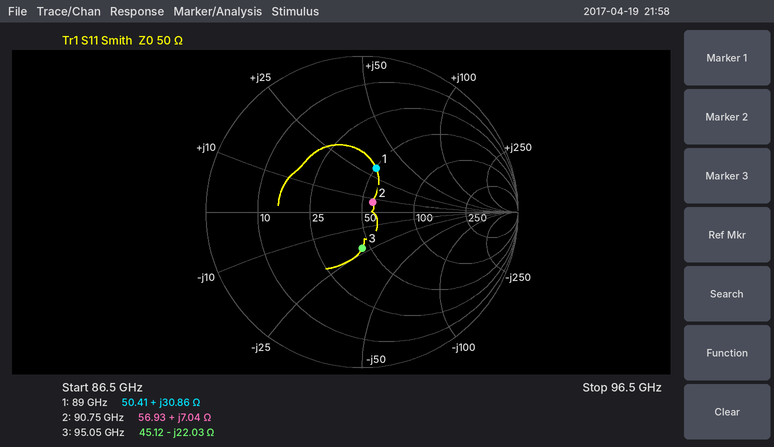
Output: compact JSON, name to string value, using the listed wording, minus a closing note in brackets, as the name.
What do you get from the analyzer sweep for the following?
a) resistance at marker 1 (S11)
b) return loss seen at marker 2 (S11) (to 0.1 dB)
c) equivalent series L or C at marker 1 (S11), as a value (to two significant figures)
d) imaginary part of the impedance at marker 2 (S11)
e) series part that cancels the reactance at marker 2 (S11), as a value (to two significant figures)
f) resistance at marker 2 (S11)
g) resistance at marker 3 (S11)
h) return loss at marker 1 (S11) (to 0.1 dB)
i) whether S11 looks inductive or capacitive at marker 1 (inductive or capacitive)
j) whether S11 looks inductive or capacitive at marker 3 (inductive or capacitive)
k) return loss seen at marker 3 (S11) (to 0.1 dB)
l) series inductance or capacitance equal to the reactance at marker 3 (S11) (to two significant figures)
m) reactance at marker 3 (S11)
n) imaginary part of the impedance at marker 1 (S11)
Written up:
{"resistance at marker 1": "50.41 Ω", "return loss seen at marker 2 (S11)": "20.7 dB", "equivalent series L or C at marker 1 (S11), as a value": "55 pH", "imaginary part of the impedance at marker 2": "+7.04 Ω", "series part that cancels the reactance at marker 2 (S11), as a value": "250 fF", "resistance at marker 2": "56.93 Ω", "resistance at marker 3": "45.12 Ω", "return loss at marker 1 (S11)": "10.6 dB", "whether S11 looks inductive or capacitive at marker 1": "inductive", "whether S11 looks inductive or capacitive at marker 3": "capacitive", "return loss seen at marker 3 (S11)": "12.7 dB", "series inductance or capacitance equal to the reactance at marker 3 (S11)": "76 fF", "reactance at marker 3": "-22.03 Ω", "imaginary part of the impedance at marker 1": "+30.86 Ω"}
